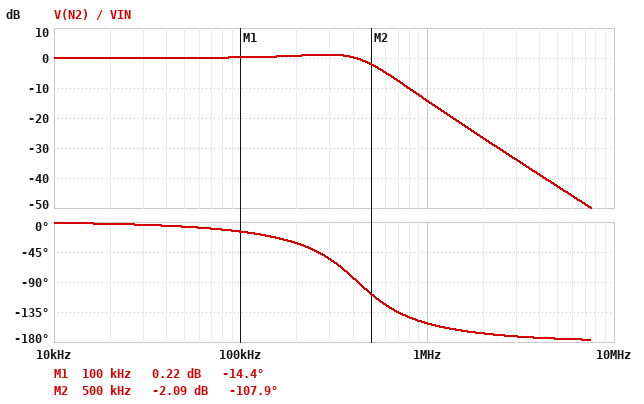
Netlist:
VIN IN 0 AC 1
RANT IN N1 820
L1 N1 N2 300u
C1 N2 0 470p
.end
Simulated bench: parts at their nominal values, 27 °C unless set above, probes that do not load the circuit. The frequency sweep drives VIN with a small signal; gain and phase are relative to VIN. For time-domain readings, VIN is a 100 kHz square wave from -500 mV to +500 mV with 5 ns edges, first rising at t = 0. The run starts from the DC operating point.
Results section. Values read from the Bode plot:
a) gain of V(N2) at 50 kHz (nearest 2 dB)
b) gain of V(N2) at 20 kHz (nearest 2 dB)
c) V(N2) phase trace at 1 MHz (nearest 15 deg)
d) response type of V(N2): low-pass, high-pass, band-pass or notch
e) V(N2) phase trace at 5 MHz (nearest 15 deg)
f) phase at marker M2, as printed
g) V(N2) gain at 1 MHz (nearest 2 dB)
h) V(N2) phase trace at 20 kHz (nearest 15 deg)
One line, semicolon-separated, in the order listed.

0 dB; 0 dB; -150 deg; low-pass; -180 deg; -107.9 deg; -14 dB; 0 deg
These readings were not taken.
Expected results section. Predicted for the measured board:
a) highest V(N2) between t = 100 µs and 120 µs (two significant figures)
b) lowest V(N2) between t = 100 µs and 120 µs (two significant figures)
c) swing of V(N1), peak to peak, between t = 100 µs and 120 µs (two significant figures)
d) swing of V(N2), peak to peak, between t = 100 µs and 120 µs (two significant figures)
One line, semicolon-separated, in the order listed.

650 mV; -650 mV; 1.2 V; 1.3 V
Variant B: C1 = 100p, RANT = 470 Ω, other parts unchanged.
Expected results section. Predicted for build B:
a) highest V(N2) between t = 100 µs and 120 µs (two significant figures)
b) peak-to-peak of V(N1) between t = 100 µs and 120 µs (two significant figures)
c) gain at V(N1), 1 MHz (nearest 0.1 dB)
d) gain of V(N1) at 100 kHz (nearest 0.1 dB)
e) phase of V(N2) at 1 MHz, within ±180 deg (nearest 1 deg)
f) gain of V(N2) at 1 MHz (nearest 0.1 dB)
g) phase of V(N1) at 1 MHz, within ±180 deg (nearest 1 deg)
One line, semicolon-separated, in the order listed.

1.2 V; 1.3 V; -5.5 dB; 0 dB; -122 deg; 9.2 dB; 58 deg
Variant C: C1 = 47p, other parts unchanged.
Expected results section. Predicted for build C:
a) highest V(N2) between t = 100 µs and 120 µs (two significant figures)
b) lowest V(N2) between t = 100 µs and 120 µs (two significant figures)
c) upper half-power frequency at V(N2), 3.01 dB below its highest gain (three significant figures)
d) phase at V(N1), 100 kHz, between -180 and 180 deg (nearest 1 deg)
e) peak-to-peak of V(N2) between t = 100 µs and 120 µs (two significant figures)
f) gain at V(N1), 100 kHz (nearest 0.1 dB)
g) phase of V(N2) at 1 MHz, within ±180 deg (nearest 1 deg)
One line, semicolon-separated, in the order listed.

1.1 V; -1.1 V; 1.51 MHz; -1 deg; 2.2 V; 0 dB; -29 deg
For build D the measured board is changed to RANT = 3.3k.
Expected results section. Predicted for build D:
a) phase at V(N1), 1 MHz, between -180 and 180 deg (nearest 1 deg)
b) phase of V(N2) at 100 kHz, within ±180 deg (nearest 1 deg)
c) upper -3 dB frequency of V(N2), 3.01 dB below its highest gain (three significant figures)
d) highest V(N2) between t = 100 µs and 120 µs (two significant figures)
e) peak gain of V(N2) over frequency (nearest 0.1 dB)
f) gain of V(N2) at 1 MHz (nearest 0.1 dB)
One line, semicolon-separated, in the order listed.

65 deg; -46 deg; 109 kHz; 470 mV; 0 dB; -20.6 dB
